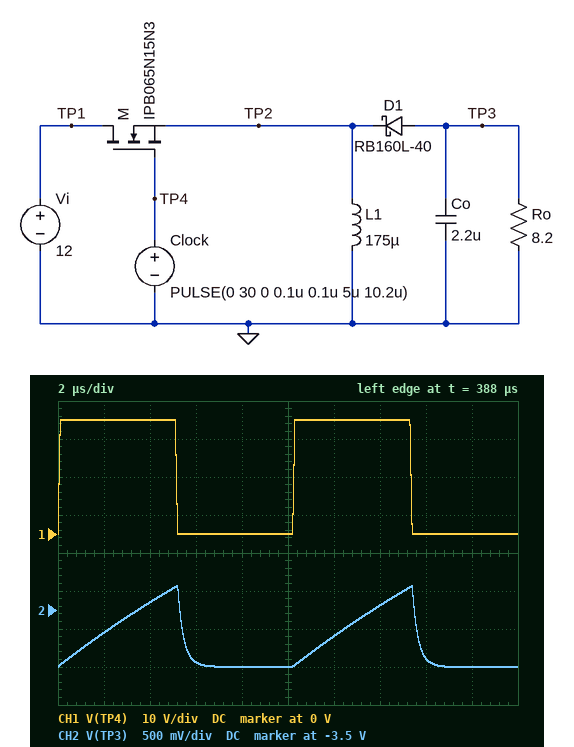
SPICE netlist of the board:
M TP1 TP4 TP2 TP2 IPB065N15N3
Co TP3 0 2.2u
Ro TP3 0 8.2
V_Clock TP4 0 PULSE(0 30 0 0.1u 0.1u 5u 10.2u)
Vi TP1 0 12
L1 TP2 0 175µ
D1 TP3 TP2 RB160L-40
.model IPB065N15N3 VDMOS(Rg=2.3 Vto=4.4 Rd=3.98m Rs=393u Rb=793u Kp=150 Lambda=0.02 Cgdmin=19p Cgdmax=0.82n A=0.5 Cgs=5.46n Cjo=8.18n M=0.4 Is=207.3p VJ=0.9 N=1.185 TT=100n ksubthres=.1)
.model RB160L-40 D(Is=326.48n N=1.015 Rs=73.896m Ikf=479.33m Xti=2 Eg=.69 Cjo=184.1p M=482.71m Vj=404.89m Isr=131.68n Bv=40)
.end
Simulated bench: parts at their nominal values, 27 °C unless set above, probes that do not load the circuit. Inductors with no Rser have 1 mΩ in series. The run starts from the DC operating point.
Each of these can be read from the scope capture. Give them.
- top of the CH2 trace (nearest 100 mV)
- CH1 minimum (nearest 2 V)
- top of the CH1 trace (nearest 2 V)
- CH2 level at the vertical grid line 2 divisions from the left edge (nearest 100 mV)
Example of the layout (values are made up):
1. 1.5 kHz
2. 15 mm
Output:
1. -3.2 V
2. 0 V
3. 30 V
4. -3.4 V
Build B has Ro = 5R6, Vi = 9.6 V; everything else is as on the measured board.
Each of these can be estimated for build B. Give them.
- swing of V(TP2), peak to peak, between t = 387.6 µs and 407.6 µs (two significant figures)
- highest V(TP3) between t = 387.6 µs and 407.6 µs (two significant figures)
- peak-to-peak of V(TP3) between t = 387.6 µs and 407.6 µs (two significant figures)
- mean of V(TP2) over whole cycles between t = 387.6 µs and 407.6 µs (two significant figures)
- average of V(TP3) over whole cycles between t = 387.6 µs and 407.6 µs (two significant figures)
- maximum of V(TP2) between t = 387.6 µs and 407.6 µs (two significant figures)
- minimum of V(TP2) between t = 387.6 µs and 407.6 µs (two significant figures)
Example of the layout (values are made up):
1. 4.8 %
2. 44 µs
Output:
1. 14 V
2. -2.7 V
3. 1.4 V
4. 2.6 V
5. -3.7 V
6. 9.6 V
7. -4.6 V
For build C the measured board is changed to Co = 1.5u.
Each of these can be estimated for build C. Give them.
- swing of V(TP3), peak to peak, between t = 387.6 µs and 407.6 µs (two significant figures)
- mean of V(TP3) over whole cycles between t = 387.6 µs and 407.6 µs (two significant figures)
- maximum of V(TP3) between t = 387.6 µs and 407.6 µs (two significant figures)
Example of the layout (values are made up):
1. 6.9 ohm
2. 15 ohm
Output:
1. 1.5 V
2. -3.8 V
3. -2.8 V
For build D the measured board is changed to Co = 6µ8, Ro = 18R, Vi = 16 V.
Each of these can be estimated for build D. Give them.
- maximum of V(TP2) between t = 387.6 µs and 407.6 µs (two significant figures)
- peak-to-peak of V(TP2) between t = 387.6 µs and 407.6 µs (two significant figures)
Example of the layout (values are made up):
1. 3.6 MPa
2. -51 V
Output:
1. 16 V
2. 21 V
